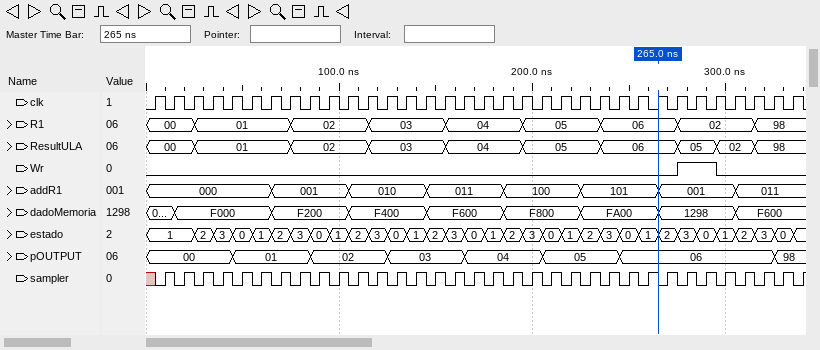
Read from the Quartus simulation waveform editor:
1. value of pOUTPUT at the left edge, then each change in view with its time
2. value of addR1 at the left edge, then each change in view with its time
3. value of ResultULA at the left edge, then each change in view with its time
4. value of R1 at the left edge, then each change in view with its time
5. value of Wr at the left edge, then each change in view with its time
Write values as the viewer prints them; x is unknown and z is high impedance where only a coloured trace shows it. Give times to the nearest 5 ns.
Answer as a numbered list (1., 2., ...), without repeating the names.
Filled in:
1. 00, 01 at 45 ns, 02 at 85 ns, 03 at 125 ns, 04 at 165 ns, 05 at 205 ns, 06 at 245 ns, 98 at 325 ns
2. 000, 001 at 65 ns, 010 at 105 ns, 011 at 145 ns, 100 at 185 ns, 101 at 225 ns, 001 at 265 ns, 011 at 305 ns
3. 00, 01 at 25 ns, 02 at 75 ns, 03 at 115 ns, 04 at 155 ns, 05 at 195 ns, 06 at 235 ns, 05 at 275 ns, 02 at 295 ns, 98 at 315 ns
4. 00, 01 at 25 ns, 02 at 75 ns, 03 at 115 ns, 04 at 155 ns, 05 at 195 ns, 06 at 235 ns, 02 at 275 ns, 98 at 315 ns
5. 0, 1 at 275 ns, 0 at 295 ns
